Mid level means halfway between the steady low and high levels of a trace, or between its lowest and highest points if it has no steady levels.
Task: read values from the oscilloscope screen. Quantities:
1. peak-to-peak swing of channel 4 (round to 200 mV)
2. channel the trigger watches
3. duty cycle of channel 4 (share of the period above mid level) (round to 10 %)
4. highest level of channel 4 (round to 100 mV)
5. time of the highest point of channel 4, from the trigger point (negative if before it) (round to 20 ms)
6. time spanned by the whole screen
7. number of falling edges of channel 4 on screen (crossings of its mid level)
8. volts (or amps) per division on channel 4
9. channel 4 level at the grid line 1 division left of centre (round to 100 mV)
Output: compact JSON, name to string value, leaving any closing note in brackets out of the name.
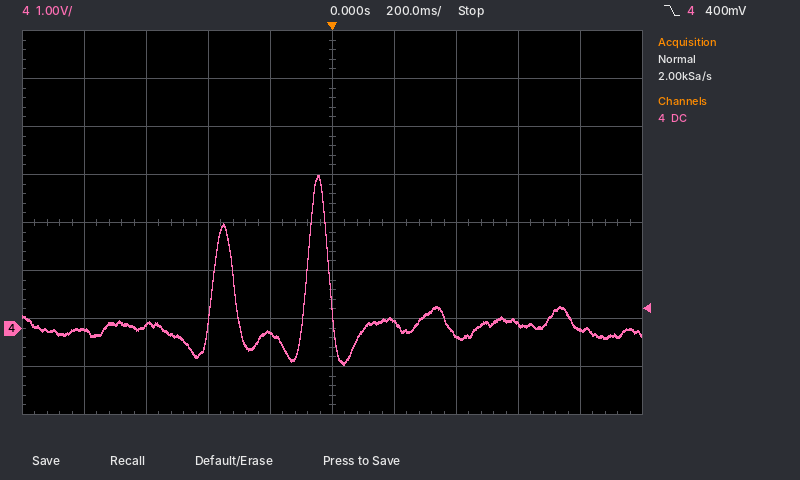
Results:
{"peak-to-peak swing of channel 4": "4.0 V", "channel the trigger watches": "channel 4", "duty cycle of channel 4 (share of the period above mid level)": "20 %", "highest level of channel 4": "3.2 V", "time of the highest point of channel 4, from the trigger point (negative if before it)": "-40 ms", "time spanned by the whole screen": "2 s", "number of falling edges of channel 4 on screen": "2", "volts (or amps) per division on channel 4": "1 V", "channel 4 level at the grid line 1 division left of centre": "-100 mV"}
